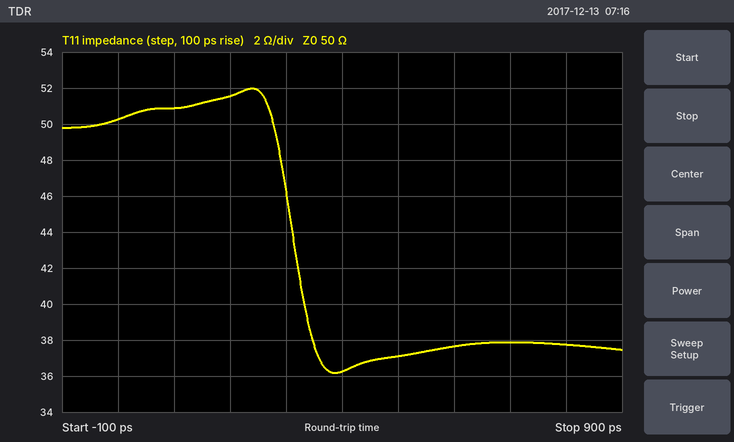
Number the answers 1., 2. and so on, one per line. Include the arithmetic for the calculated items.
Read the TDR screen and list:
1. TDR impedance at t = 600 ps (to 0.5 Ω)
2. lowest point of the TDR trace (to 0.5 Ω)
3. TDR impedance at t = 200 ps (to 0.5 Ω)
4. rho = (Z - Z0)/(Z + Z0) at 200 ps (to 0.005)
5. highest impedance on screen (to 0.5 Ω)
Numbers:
1. 37.5 Ω
2. 36.0 Ω
3. 51.5 Ω
4. (51.5 − 50)/(51.5 + 50) ≈ +0.015
5. 52.0 Ω
